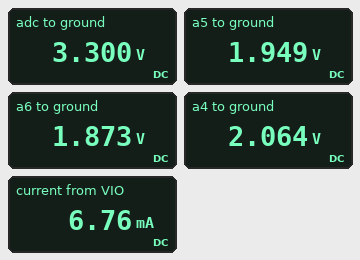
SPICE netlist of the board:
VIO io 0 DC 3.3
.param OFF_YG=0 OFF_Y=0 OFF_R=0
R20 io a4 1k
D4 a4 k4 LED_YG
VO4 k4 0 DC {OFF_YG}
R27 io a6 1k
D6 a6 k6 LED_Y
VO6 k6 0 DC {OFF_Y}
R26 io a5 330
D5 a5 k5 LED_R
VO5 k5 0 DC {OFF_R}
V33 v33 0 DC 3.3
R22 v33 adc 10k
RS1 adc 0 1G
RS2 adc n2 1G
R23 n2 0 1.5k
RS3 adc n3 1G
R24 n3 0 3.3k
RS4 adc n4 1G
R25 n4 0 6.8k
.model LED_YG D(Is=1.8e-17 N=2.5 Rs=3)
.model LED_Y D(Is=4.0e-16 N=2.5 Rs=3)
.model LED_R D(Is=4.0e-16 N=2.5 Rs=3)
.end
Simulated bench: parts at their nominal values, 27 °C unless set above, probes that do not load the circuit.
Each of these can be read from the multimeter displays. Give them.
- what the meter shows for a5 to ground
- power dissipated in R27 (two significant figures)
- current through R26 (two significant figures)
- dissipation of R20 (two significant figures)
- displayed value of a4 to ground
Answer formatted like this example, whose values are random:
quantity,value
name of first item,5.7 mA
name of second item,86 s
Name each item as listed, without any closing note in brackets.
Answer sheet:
quantity,value
what the meter shows for a5 to ground,1.949 V
power dissipated in R27,2.0 mW
current through R26,4.1 mA
dissipation of R20,1.5 mW
displayed value of a4 to ground,2.064 V
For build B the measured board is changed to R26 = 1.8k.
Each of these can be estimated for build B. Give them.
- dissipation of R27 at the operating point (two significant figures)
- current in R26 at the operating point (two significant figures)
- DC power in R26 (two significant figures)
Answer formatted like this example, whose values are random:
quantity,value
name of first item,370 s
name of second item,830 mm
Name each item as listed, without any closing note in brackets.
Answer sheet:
quantity,value
dissipation of R27 at the operating point,2.0 mW
current in R26 at the operating point,810 µA
DC power in R26,1.2 mW
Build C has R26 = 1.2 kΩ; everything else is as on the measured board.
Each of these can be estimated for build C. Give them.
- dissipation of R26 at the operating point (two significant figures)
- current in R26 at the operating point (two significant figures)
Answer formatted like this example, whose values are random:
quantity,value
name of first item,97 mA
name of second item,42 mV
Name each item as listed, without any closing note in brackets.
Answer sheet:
quantity,value
dissipation of R26 at the operating point,1.7 mW
current in R26 at the operating point,1.2 mA
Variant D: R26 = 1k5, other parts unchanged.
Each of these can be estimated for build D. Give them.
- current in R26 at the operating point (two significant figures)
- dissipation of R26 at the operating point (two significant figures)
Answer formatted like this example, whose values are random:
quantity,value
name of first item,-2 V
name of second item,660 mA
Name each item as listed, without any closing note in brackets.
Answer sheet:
quantity,value
current in R26 at the operating point,970 µA
dissipation of R26 at the operating point,1.4 mW
